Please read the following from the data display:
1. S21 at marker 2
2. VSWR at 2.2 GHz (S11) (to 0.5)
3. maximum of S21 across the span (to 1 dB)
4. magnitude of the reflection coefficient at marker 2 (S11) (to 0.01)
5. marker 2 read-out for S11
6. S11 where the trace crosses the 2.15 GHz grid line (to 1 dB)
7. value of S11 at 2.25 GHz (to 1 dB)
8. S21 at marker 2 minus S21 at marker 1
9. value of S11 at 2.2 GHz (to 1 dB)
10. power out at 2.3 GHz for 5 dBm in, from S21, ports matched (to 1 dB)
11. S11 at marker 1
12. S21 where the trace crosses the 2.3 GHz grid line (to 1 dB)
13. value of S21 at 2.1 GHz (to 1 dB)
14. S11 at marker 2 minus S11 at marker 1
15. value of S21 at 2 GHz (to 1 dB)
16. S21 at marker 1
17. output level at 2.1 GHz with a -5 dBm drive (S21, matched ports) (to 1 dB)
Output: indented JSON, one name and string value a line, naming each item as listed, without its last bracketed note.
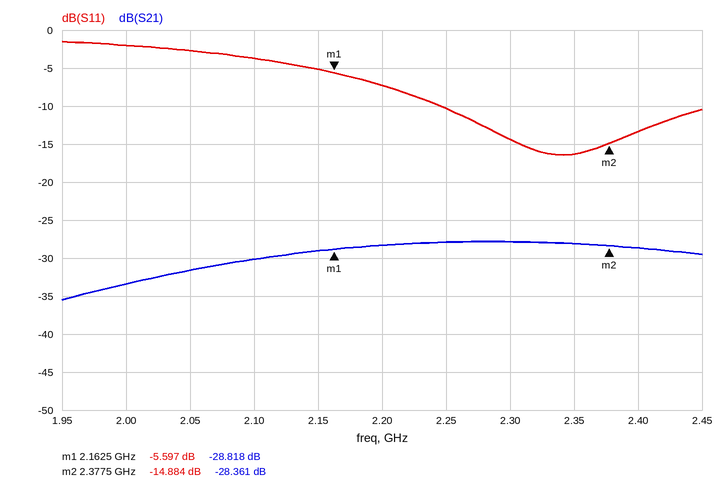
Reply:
{
  "S21 at marker 2": "-28.361 dB",
  "VSWR at 2.2 GHz (S11)": "2.5",
  "maximum of S21 across the span": "-28 dB",
  "magnitude of the reflection coefficient at marker 2 (S11)": "0.18",
  "marker 2 read-out for S11": "-14.884 dB",
  "S11 where the trace crosses the 2.15 GHz grid line": "-5 dB",
  "value of S11 at 2.25 GHz": "-10 dB",
  "S21 at marker 2 minus S21 at marker 1": "0.457 dB",
  "value of S11 at 2.2 GHz": "-7 dB",
  "power out at 2.3 GHz for 5 dBm in, from S21, ports matched": "-23 dBm",
  "S11 at marker 1": "-5.597 dB",
  "S21 where the trace crosses the 2.3 GHz grid line": "-28 dB",
  "value of S21 at 2.1 GHz": "-30 dB",
  "S11 at marker 2 minus S11 at marker 1": "-9.287 dB",
  "value of S21 at 2 GHz": "-33 dB",
  "S21 at marker 1": "-28.818 dB",
  "output level at 2.1 GHz with a -5 dBm drive (S21, matched ports)": "-35 dBm"
}
